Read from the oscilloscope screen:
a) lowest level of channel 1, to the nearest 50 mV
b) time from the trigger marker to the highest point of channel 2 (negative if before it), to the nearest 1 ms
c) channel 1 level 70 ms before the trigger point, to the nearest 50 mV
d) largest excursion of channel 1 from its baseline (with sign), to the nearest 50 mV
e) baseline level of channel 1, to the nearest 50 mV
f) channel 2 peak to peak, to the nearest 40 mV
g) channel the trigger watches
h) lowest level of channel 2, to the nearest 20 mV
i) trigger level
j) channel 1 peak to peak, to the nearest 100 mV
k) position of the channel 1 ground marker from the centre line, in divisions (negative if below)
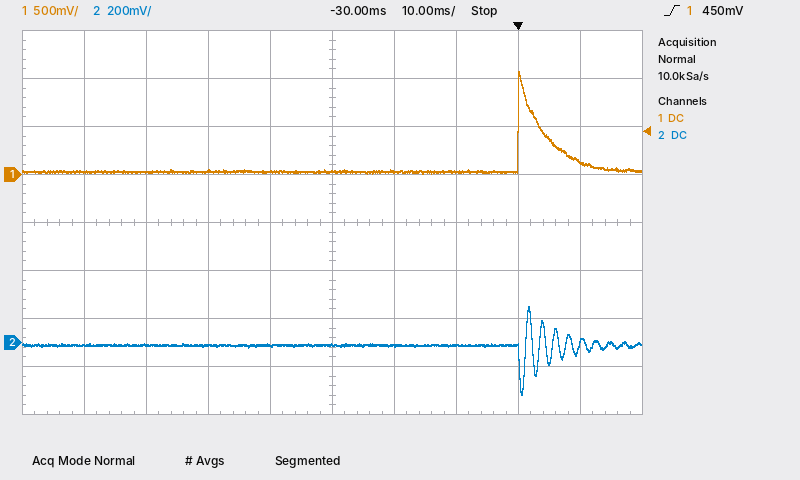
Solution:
0 mV
+2 ms
50 mV
+1.05 V
50 mV
360 mV
channel 1
-220 mV
450 mV
1.10 V
+1.0 div
